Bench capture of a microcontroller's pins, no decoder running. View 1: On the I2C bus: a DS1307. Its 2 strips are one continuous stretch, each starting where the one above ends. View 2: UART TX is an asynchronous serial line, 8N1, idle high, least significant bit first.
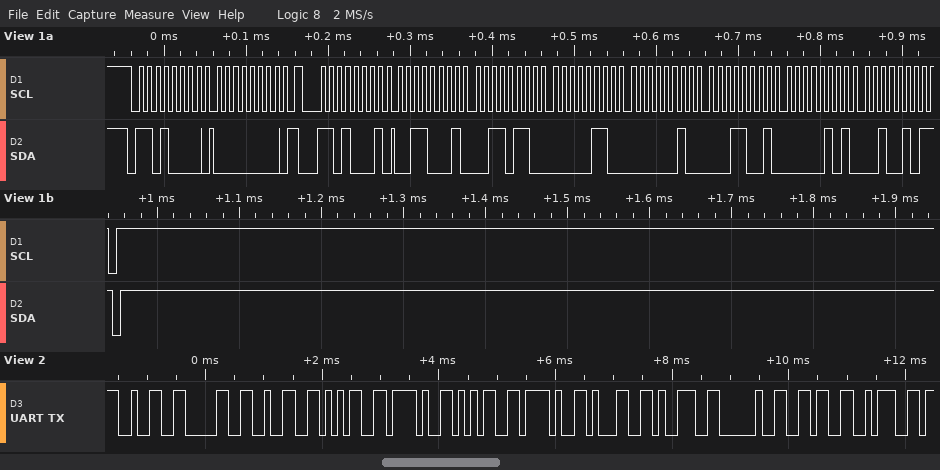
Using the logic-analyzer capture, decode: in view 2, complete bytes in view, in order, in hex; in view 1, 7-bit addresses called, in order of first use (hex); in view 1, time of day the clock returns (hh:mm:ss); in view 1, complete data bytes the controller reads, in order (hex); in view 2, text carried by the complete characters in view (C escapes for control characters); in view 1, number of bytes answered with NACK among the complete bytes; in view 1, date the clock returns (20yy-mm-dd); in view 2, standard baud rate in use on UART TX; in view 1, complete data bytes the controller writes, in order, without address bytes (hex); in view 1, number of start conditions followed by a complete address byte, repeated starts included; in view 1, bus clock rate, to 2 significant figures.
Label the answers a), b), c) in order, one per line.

a) 32 30 32 35 2F 35 2F 31 39 20 36 3A
b) 0x68
c) 06:36:31
d) 31 36 06 02 19 05 25
e) "2025/5/19 6:"
f) 1
g) 2025-05-19
h) 9600 baud
i) 00
j) 2
k) 100 kHz
